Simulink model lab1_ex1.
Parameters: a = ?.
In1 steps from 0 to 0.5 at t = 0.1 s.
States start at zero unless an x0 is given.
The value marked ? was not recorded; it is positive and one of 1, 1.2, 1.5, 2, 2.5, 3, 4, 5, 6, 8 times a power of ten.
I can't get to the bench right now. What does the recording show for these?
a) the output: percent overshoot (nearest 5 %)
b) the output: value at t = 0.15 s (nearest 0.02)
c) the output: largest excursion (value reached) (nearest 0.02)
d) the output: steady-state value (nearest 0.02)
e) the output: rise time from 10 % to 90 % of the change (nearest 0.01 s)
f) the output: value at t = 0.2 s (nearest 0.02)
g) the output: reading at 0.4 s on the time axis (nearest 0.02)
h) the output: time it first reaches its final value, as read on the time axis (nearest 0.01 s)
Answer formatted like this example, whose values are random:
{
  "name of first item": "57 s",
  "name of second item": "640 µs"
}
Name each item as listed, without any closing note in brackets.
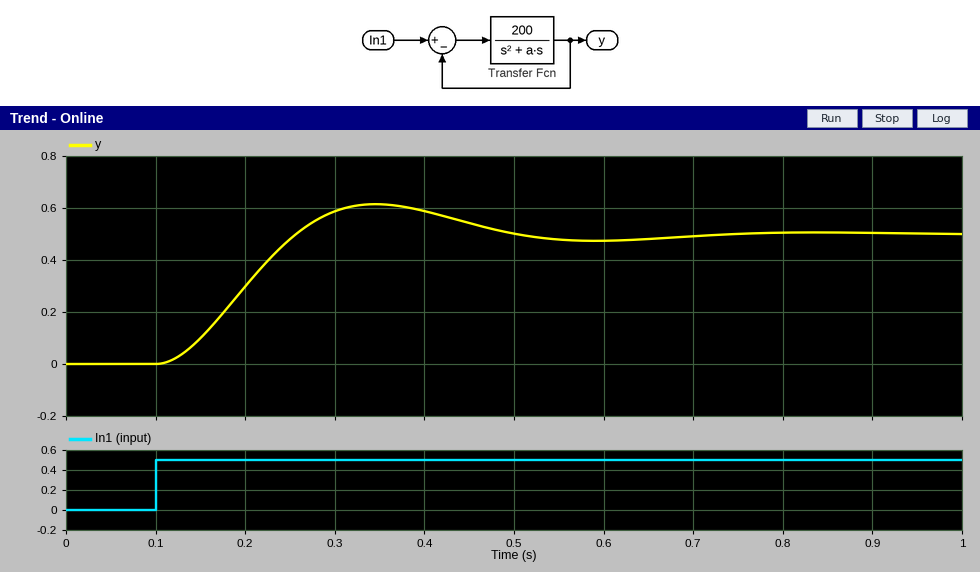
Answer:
{
  "the output: percent overshoot": "25 %",
  "the output: value at t = 0.15 s": "0.10",
  "the output: largest excursion (value reached)": "0.62",
  "the output: steady-state value": "0.50",
  "the output: rise time from 10 % to 90 % of the change": "0.11 s",
  "the output: value at t = 0.2 s": "0.30",
  "the output: reading at 0.4 s on the time axis": "0.58",
  "the output: time it first reaches its final value, as read on the time axis": "0.26 s"
}
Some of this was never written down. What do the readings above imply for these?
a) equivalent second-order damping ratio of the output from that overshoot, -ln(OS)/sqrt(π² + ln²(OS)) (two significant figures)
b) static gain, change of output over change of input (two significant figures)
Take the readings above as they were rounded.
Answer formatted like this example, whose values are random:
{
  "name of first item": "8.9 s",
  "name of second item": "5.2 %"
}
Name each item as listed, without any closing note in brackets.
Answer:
{
  "equivalent second-order damping ratio of the output from that overshoot, -ln(OS)/sqrt(π² + ln²(OS))": "0.40",
  "static gain, change of output over change of input": "1.0"
}
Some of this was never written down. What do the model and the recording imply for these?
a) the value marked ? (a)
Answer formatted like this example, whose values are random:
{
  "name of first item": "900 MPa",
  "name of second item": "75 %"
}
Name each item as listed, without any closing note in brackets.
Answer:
{
  "the value marked ?": "12"
}
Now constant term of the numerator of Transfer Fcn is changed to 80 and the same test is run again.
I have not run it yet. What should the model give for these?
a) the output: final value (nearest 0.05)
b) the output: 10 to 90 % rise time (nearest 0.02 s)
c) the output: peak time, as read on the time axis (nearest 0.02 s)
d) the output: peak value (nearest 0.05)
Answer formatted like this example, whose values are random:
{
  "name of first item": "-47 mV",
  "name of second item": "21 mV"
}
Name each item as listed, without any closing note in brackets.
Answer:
{
  "the output: final value": "0.50",
  "the output: 10 to 90 % rise time": "0.22 s",
  "the output: peak time, as read on the time axis": "0.58 s",
  "the output: peak value": "0.55"
}
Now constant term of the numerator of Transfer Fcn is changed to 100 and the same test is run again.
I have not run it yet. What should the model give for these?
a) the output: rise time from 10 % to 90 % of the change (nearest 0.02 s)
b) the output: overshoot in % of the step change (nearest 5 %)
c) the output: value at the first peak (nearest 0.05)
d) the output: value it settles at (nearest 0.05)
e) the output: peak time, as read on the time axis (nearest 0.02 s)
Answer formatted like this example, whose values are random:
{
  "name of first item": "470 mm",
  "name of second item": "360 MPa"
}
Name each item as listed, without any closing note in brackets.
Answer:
{
  "the output: rise time from 10 % to 90 % of the change": "0.18 s",
  "the output: overshoot in % of the step change": "10 %",
  "the output: value at the first peak": "0.55",
  "the output: value it settles at": "0.50",
  "the output: peak time, as read on the time axis": "0.50 s"
}
